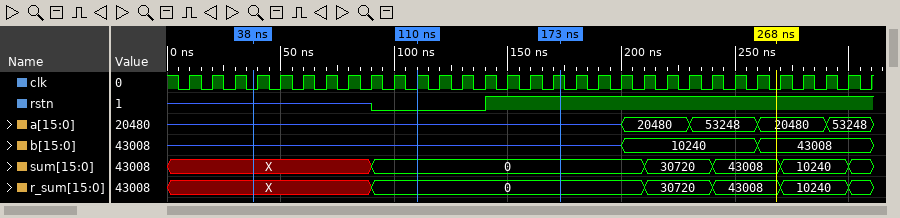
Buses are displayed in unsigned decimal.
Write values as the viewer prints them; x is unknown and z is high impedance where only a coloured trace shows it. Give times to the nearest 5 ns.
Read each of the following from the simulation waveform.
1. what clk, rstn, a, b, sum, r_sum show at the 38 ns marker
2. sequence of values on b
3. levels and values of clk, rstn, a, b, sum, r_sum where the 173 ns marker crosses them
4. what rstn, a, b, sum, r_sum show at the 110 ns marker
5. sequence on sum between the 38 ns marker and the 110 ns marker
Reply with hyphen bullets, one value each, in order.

- clk=0, rstn=z, a=z, b=z, sum=X, r_sum=X
- z, 10240, 43008
- clk=1, rstn=1, a=z, b=z, sum=0, r_sum=0
- rstn=0, a=z, b=z, sum=0, r_sum=0
- X, 0
